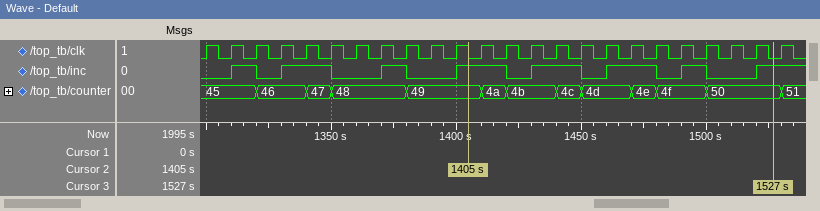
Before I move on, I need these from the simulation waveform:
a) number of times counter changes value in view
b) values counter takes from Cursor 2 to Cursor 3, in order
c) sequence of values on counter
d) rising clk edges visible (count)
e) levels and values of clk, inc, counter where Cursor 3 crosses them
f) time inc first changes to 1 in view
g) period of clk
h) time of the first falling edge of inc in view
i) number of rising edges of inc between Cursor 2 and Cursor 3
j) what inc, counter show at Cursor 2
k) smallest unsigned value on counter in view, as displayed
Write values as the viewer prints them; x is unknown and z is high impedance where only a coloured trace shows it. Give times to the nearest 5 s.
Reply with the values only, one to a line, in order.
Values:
12
49, 4a, 4b, 4c, 4d, 4e, 4f, 50
45, 46, 47, 48, 49, 4a, 4b, 4c, 4d, 4e, 4f, 50, 51
24
clk=0, inc=1, counter=50
1310 s
10 s
1320 s
4
inc=1, counter=49
45
